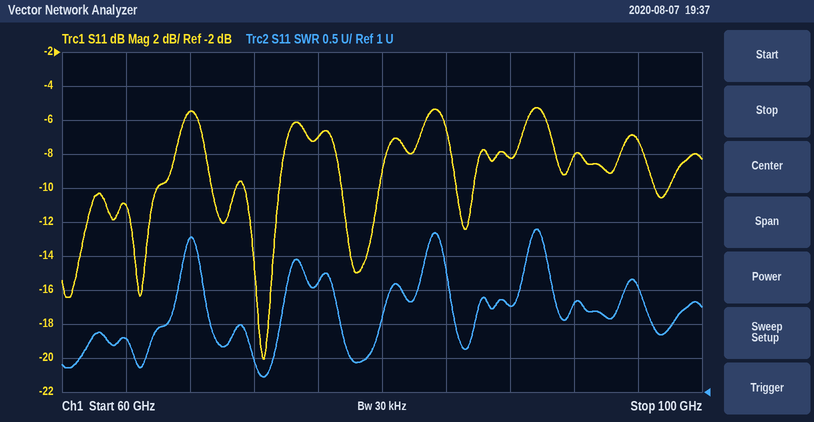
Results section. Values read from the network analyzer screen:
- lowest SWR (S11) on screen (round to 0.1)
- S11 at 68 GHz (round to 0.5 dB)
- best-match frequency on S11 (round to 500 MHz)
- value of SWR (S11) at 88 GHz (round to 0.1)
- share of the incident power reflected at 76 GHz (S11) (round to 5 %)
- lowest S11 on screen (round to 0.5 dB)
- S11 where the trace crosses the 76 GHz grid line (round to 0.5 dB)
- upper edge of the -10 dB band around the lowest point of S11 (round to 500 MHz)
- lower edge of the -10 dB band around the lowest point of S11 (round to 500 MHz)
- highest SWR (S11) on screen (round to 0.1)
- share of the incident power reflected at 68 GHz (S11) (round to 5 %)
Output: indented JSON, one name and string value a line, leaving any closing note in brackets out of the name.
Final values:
{
  "lowest SWR (S11) on screen": "1.2",
  "S11 at 68 GHz": "-5.5 dB",
  "best-match frequency on S11": "72.5 GHz",
  "value of SWR (S11) at 88 GHz": "2.3",
  "share of the incident power reflected at 76 GHz (S11)": "20 %",
  "lowest S11 on screen": "-20.0 dB",
  "S11 where the trace crosses the 76 GHz grid line": "-7.0 dB",
  "upper edge of the -10 dB band around the lowest point of S11": "73.5 GHz",
  "lower edge of the -10 dB band around the lowest point of S11": "71.5 GHz",
  "highest SWR (S11) on screen": "3.4",
  "share of the incident power reflected at 68 GHz (S11)": "30 %"
}
